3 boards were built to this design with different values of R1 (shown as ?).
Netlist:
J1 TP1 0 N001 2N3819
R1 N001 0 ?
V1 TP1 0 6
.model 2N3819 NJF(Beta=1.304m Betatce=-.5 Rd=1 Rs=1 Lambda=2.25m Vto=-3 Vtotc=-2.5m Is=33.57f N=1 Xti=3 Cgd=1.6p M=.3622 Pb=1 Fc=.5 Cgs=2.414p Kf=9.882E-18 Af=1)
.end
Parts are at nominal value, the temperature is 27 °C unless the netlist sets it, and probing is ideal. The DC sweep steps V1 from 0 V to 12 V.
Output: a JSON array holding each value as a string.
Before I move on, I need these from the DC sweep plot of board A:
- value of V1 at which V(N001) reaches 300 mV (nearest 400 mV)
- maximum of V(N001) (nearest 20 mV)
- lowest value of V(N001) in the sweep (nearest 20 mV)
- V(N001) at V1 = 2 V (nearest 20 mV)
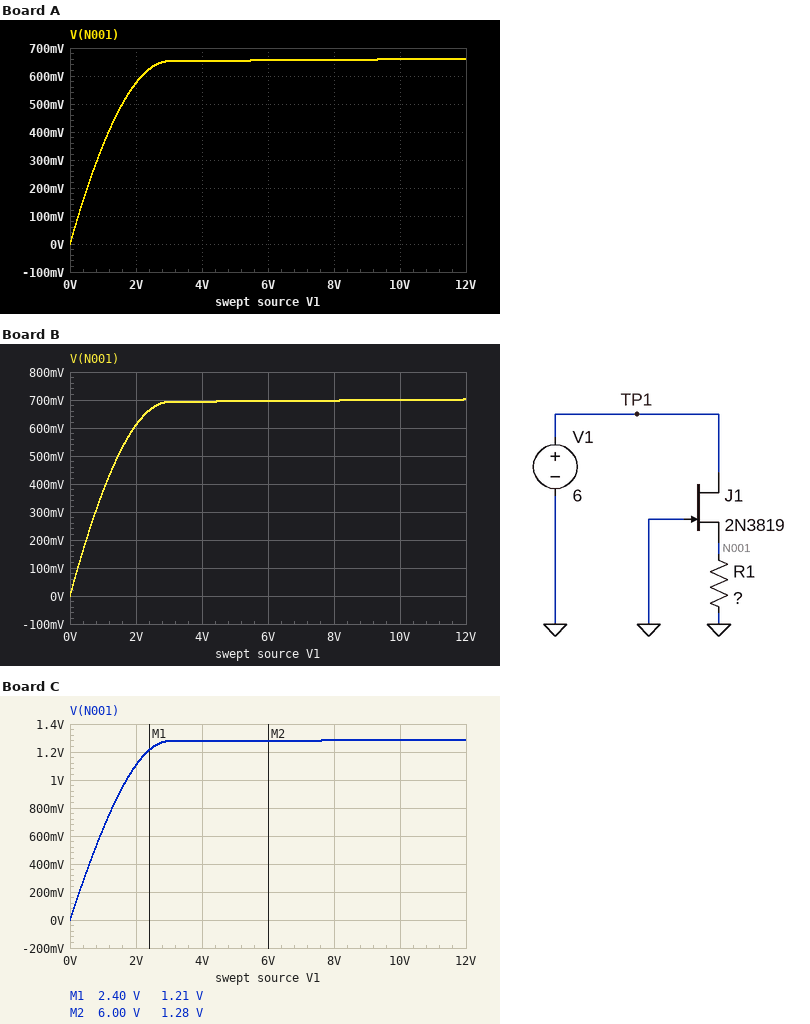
["800 mV", "660 mV", "0 V", "580 mV"]
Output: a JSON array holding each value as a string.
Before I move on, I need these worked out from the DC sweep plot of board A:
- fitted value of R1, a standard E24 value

["91 Ω"]
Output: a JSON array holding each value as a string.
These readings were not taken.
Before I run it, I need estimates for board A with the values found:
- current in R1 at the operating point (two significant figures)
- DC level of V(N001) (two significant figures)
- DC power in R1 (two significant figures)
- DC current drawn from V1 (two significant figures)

["7.2 mA", "660 mV", "4.7 mW", "7.2 mA"]
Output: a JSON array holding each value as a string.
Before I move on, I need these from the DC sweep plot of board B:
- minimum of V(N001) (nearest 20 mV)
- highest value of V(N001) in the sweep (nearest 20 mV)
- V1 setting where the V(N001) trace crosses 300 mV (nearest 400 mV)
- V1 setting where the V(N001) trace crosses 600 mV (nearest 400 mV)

["0 V", "700 mV", "800 mV", "2.0 V"]
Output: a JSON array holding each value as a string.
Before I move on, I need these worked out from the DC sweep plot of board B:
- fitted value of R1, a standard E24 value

["100 Ω"]
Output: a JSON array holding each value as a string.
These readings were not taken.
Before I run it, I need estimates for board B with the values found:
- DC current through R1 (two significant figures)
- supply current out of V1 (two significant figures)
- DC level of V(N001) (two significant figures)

["7.0 mA", "7.0 mA", "700 mV"]
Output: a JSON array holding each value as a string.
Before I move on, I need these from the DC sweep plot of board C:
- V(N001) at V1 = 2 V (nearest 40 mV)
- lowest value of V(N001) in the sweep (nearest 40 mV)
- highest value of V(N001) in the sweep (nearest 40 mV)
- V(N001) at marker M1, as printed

["1.12 V", "0 V", "1.28 V", "1.21 V"]
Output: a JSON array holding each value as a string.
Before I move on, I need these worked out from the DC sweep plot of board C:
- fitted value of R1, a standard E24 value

["330 Ω"]
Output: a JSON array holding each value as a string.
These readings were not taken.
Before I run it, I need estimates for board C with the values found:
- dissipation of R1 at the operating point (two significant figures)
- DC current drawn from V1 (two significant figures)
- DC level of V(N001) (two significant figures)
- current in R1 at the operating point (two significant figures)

["5.0 mW", "3.9 mA", "1.3 V", "3.9 mA"]
